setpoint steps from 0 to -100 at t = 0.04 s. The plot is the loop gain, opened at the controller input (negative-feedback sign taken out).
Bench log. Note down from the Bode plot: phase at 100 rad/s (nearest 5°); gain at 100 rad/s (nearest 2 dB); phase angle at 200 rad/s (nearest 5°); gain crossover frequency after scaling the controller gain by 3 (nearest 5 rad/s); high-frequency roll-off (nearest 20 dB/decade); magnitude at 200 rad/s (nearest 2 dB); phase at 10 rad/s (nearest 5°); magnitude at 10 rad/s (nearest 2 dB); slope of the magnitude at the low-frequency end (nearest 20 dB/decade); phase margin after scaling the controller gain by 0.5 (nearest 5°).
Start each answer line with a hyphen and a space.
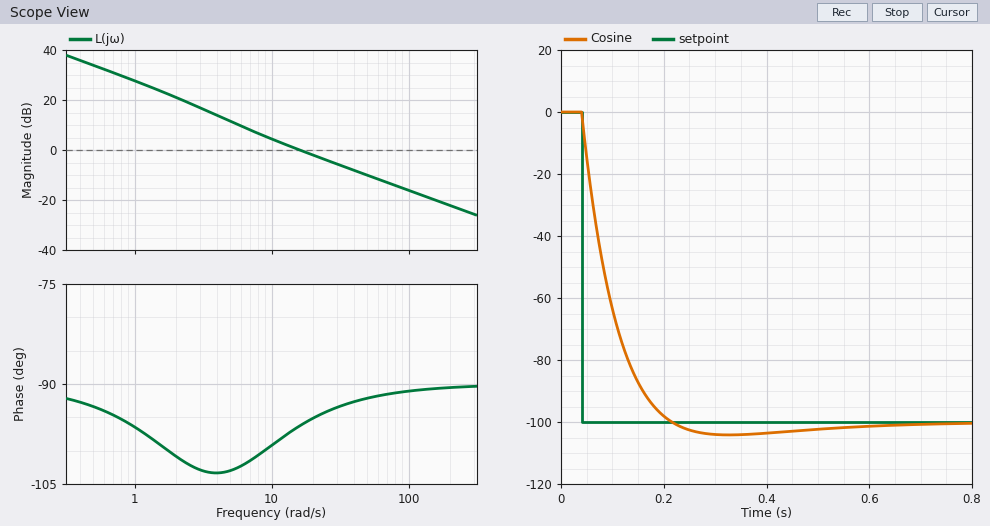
- -90°
- -16 dB
- -90°
- 45 rad/s
- -20 dB/decade
- -22 dB
- -100°
- 4 dB
- -20 dB/decade
- 80°
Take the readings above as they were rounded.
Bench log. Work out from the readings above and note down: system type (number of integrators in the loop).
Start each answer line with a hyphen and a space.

- 1
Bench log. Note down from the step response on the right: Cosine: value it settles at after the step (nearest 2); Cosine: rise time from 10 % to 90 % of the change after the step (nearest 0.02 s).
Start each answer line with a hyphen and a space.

- -100
- 0.12 s
